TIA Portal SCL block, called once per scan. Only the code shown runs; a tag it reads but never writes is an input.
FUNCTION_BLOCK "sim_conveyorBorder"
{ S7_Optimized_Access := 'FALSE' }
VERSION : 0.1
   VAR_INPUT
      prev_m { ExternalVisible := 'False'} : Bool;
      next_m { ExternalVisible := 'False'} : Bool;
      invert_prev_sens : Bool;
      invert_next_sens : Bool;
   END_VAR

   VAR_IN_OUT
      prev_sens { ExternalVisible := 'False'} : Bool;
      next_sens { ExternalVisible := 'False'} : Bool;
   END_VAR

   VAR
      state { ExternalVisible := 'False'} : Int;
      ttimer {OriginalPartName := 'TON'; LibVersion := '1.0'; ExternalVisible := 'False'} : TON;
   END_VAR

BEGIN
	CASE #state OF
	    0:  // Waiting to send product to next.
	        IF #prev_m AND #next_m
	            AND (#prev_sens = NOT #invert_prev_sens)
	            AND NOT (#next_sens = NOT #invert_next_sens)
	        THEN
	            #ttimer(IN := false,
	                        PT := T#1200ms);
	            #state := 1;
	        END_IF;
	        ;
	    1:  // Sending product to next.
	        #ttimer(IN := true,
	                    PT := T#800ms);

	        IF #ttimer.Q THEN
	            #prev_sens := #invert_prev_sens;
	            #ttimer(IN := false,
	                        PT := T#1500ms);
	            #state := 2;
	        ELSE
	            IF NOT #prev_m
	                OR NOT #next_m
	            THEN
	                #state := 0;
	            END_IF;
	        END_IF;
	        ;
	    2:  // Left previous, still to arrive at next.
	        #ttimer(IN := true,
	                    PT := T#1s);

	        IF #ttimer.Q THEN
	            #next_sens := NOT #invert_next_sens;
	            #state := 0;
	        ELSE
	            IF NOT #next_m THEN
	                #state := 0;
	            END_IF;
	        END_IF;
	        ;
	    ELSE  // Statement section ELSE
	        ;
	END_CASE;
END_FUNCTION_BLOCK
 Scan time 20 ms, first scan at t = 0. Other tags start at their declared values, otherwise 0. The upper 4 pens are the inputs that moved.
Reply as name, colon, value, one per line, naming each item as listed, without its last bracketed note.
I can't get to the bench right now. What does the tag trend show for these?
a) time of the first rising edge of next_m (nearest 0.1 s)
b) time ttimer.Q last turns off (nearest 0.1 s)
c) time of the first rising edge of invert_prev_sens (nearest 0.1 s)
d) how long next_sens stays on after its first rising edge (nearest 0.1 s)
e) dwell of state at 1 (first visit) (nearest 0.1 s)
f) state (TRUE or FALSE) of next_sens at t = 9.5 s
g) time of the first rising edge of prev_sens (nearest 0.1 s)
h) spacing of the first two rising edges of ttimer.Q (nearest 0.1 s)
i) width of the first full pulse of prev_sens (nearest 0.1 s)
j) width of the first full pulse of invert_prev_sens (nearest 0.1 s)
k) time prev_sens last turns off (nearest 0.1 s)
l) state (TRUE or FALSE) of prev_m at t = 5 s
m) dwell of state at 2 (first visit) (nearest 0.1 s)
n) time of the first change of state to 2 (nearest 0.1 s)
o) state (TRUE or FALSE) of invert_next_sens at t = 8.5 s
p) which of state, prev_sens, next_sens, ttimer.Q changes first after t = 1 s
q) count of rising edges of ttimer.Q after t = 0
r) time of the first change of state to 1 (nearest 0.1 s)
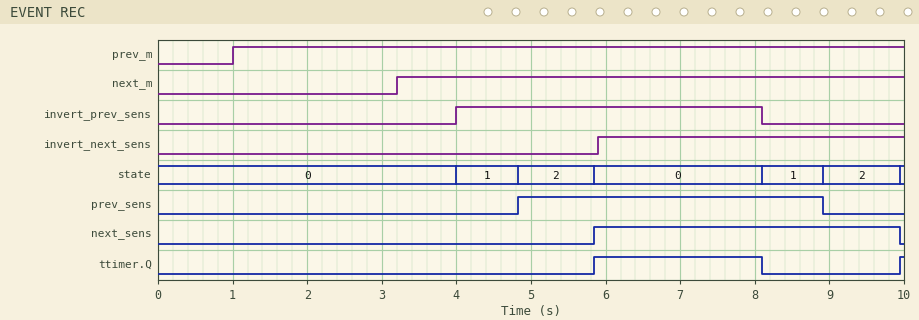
time of the first rising edge of next_m: 3.2 s
time ttimer.Q last turns off: 8.1 s
time of the first rising edge of invert_prev_sens: 4.0 s
how long next_sens stays on after its first rising edge: 4.1 s
dwell of state at 1 (first visit): 0.8 s
state (TRUE or FALSE) of next_sens at t = 9.5 s: TRUE
time of the first rising edge of prev_sens: 4.8 s
spacing of the first two rising edges of ttimer.Q: 4.1 s
width of the first full pulse of prev_sens: 4.1 s
width of the first full pulse of invert_prev_sens: 4.1 s
time prev_sens last turns off: 8.9 s
state (TRUE or FALSE) of prev_m at t = 5 s: TRUE
dwell of state at 2 (first visit): 1.0 s
time of the first change of state to 2: 4.8 s
state (TRUE or FALSE) of invert_next_sens at t = 8.5 s: TRUE
which of state, prev_sens, next_sens, ttimer.Q changes first after t = 1 s: state
count of rising edges of ttimer.Q after t = 0: 2
time of the first change of state to 1: 4.0 s
